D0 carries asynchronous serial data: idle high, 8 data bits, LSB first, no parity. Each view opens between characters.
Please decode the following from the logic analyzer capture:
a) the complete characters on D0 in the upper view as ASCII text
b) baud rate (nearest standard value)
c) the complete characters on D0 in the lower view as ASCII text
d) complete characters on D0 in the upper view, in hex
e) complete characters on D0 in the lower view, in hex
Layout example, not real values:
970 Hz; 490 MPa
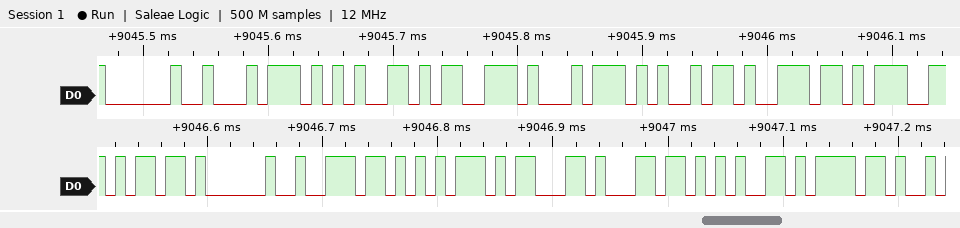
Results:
" testin"; 115200 baud; "m nucleo"; 20, 74, 65, 73, 74, 69, 6E; 6D, 20, 6E, 75, 63, 6C, 65, 6F
